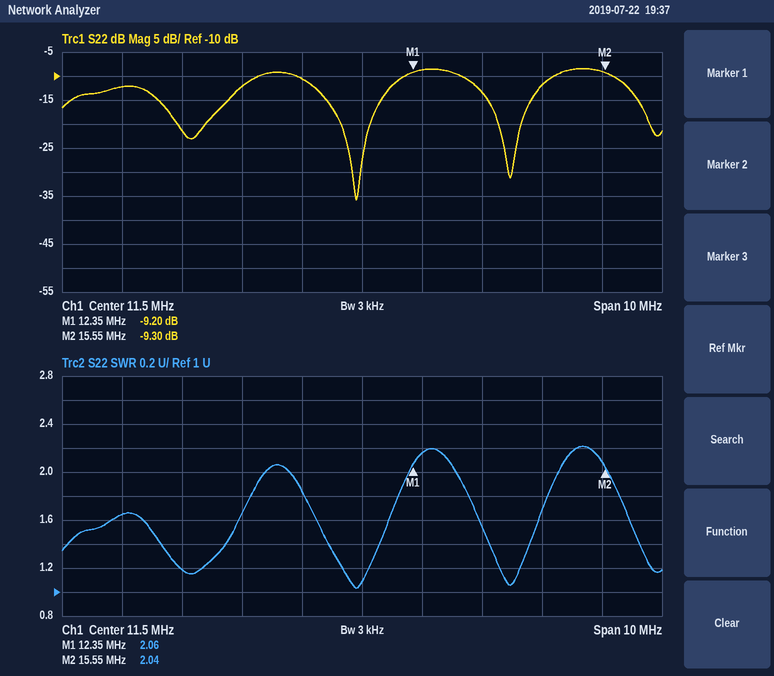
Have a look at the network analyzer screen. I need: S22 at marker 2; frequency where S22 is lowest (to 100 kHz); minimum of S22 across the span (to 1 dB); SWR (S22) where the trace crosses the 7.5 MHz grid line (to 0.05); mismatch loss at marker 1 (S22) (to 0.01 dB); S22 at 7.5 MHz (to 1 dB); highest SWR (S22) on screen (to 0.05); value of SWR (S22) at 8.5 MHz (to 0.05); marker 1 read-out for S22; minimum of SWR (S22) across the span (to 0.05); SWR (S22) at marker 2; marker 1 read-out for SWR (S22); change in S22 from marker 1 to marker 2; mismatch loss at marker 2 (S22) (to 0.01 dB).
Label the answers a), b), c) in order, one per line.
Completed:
a) -9.30 dB
b) 11.4 MHz
c) -36 dB
d) 1.65
e) 0.56 dB
f) -12 dB
g) 2.20
h) 1.20
i) -9.20 dB
j) 1.05
k) 2.04
l) 2.06
m) -0.10 dB
n) 0.54 dB
